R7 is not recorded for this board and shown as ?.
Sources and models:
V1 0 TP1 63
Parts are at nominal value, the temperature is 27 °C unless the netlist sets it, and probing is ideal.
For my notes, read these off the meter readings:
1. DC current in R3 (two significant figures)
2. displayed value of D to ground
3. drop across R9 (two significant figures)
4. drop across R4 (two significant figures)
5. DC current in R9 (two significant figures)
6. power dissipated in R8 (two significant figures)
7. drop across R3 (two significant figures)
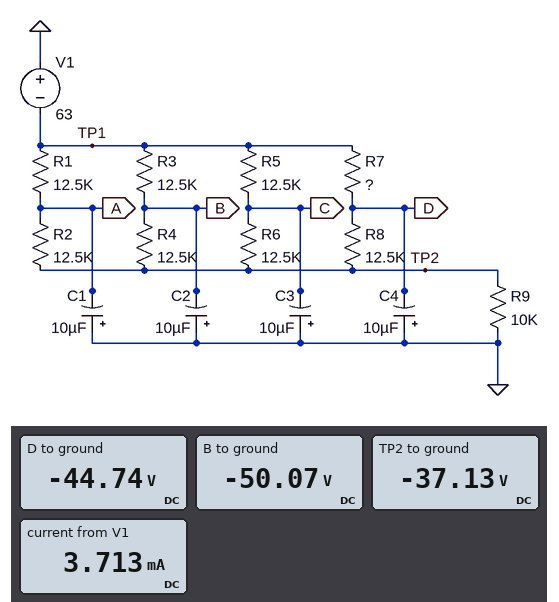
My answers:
1.0 mA
-44.74 V
37 V
13 V
3.7 mA
4.6 mW
13 V
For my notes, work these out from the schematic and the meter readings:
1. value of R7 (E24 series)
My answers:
30 kΩ
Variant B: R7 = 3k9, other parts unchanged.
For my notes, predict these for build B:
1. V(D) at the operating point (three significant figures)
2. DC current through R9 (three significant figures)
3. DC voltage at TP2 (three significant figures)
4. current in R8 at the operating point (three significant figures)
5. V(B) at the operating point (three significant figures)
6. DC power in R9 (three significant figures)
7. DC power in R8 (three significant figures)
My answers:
-57.7 V
4.06 mA
-40.6 V
1.37 mA
-51.8 V
165 mW
23.4 mW
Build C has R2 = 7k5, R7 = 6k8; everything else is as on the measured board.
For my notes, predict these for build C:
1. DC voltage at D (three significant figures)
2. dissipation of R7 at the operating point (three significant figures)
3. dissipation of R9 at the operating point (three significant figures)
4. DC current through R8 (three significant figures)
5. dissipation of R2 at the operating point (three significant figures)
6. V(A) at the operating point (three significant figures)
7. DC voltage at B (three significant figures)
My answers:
-55.1 V
9.12 mW
165 mW
1.16 mA
9.37 mW
-49.0 V
-51.8 V
